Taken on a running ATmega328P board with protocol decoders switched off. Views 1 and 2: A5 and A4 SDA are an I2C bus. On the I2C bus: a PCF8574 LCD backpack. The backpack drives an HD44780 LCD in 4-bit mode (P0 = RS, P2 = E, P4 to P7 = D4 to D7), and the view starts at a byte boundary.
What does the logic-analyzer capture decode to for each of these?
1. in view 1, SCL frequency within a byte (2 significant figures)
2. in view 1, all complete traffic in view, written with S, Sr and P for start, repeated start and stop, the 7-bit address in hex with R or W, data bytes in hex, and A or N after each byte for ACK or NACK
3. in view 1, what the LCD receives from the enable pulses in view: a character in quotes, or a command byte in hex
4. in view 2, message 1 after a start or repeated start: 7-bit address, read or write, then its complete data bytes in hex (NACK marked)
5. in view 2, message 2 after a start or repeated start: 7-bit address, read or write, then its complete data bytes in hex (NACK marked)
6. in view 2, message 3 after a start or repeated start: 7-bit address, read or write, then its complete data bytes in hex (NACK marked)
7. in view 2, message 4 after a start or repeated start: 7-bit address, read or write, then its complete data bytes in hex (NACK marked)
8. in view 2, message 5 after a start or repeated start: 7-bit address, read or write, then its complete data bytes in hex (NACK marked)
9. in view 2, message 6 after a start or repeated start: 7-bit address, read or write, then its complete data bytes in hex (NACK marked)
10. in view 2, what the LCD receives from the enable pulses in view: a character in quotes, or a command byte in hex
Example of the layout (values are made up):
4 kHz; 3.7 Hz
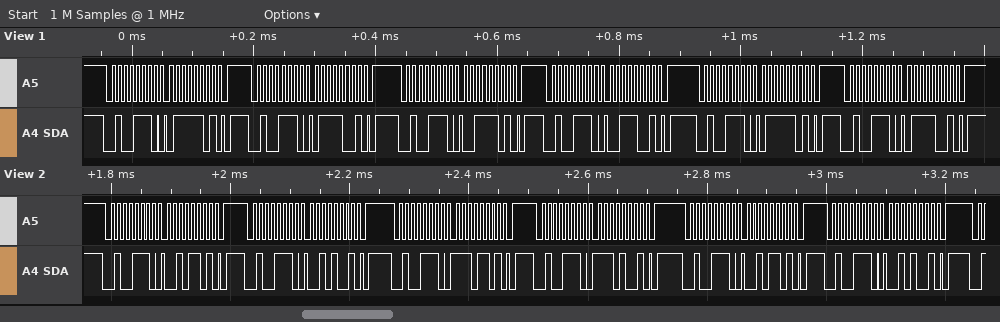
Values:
100 kHz; S 27W A 7D A P S 27W A 79 A P S 27W A 3D A P S 27W A 39 A P S 27W A 7D A P S 27W A 79 A P; 's'; 0x27 write: 2D; 0x27 write: 29; 0x27 write: ED; 0x27 write: E9; 0x27 write: 2D; 0x27 write: 29; '.'
